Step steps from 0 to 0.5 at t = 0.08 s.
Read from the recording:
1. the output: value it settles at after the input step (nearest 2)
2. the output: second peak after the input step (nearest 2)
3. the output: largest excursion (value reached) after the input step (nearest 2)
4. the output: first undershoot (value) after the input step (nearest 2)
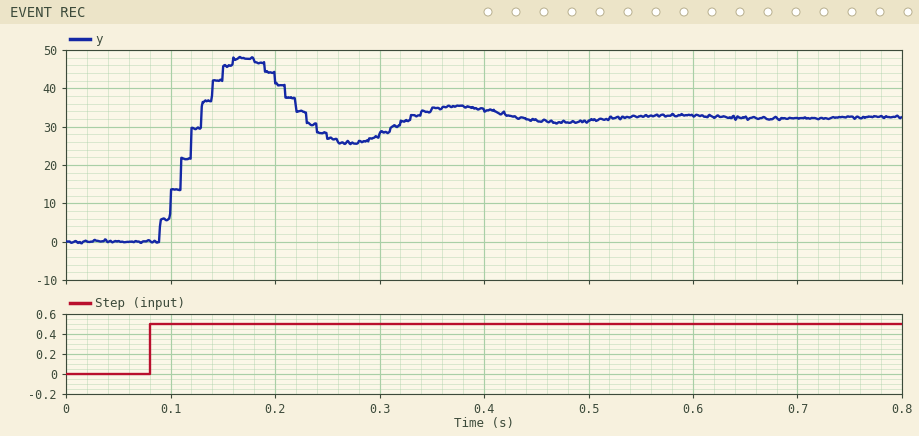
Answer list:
32
36
48
26
